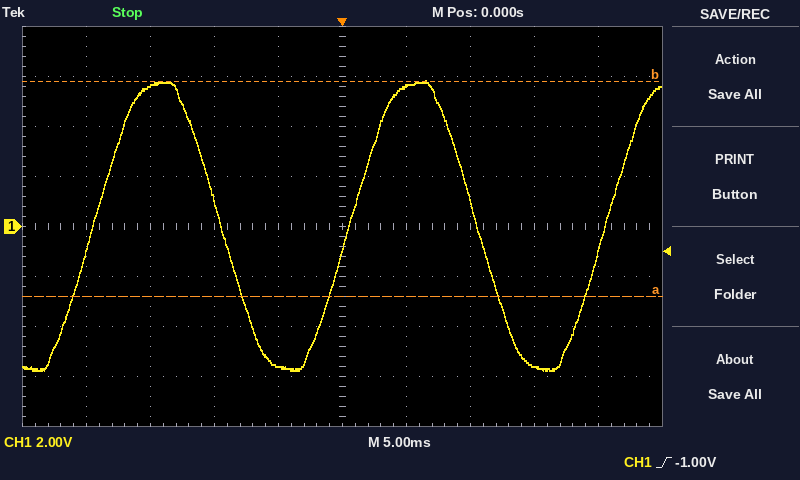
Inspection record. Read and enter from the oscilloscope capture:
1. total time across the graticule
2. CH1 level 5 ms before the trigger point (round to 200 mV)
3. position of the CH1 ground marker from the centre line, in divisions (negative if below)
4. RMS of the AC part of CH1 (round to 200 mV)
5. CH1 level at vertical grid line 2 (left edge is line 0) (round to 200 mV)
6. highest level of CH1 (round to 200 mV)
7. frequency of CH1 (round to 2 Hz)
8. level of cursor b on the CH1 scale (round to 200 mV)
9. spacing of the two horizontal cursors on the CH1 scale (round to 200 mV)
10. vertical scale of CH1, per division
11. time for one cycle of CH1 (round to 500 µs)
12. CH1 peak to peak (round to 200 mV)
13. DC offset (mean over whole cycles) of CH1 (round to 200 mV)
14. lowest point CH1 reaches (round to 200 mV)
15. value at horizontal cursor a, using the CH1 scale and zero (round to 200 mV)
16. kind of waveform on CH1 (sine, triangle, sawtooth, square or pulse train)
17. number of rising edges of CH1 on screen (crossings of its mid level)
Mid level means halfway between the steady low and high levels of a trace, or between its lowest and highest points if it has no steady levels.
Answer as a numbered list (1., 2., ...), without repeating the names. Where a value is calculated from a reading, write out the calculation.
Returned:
1. 50 ms
2. -5.6 V
3. 0.0 div
4. 11.6 V / (2√2) ≈ 4.10 V, so 4.2 V to the nearest 200 mV
5. 5.6 V
6. 5.8 V
7. 1 / 20.0 ms ≈ 50 Hz
8. 5.8 V
9. 8.6 V
10. 2 V
11. 20.0 ms
12. 5.8 V − (-5.8 V) = 11.6 V
13. (5.8 V + (-5.8 V)) / 2 ≈ 0.0 V
14. -5.8 V
15. -2.8 V
16. sine
17. 3
